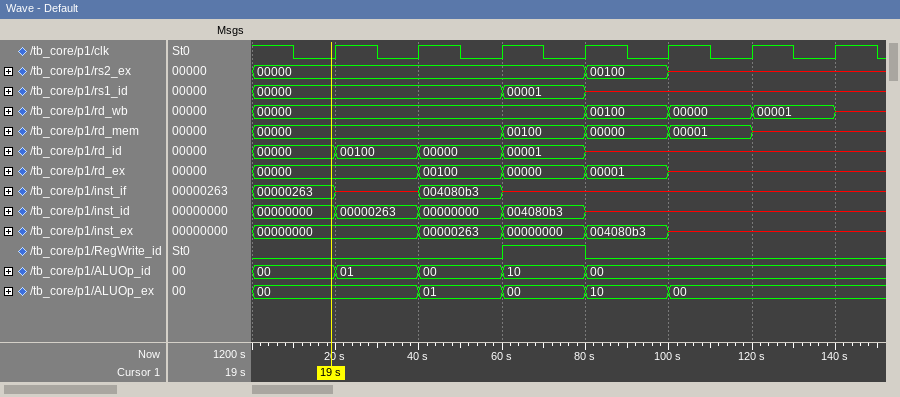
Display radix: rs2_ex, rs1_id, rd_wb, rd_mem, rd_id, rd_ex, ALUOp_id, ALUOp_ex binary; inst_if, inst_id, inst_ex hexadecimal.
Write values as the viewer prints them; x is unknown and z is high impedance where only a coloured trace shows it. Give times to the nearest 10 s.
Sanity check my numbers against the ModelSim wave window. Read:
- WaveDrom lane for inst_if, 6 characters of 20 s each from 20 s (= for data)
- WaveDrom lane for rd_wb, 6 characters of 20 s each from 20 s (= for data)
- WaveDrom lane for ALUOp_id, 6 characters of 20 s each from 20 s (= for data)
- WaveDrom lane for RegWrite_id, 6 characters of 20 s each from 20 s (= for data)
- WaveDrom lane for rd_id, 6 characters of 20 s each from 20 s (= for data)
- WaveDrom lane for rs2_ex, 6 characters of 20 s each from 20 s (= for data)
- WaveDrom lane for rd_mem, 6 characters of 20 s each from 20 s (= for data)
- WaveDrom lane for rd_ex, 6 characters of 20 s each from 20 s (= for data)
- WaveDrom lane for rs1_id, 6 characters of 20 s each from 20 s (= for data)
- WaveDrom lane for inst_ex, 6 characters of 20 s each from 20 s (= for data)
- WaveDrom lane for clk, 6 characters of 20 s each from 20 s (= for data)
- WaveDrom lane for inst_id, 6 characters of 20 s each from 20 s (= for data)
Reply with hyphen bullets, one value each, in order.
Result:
- {name: 'inst_if', wave: 'x=x...', data: '004080b3'}
- {name: 'rd_wb', wave: '=..===', data: '00000 00100 00000 00001'}
- {name: 'ALUOp_id', wave: '====..', data: '01 00 10 00'}
- {name: 'RegWrite_id', wave: '0.10..'}
- {name: 'rd_id', wave: '===x..', data: '00100 00000 00001'}
- {name: 'rs2_ex', wave: '=..=x.', data: '00000 00100'}
- {name: 'rd_mem', wave: '=.===x', data: '00000 00100 00000 00001'}
- {name: 'rd_ex', wave: '====x.', data: '00000 00100 00000 00001'}
- {name: 'rs1_id', wave: '=.=x..', data: '00000 00001'}
- {name: 'inst_ex', wave: '====x.', data: '00000000 00000263 00000000 004080b3'}
- {name: 'clk', wave: 'p.....'}
- {name: 'inst_id', wave: '===x..', data: '00000263 00000000 004080b3'}
